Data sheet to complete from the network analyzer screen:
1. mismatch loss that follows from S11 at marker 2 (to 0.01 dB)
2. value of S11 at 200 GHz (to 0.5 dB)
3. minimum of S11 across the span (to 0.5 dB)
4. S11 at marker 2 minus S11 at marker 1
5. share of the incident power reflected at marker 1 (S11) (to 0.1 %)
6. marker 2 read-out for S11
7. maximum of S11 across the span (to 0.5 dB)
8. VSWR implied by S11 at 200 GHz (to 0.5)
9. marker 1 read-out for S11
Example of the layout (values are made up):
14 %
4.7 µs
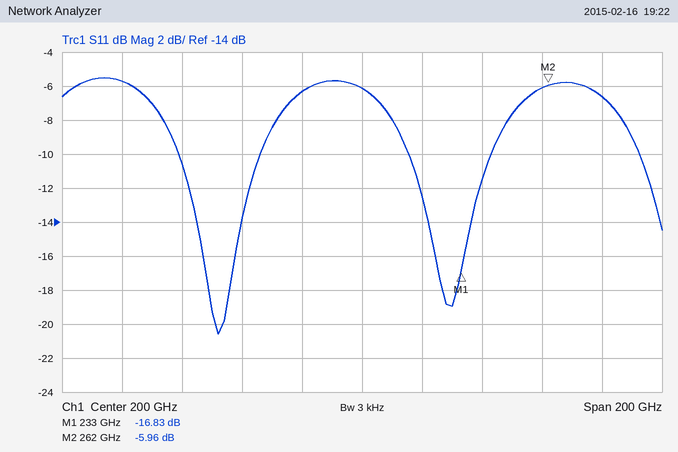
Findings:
1.27 dB
-6.0 dB
-20.5 dB
10.87 dB
2.1 %
-5.96 dB
-5.5 dB
3.0
-16.83 dB
